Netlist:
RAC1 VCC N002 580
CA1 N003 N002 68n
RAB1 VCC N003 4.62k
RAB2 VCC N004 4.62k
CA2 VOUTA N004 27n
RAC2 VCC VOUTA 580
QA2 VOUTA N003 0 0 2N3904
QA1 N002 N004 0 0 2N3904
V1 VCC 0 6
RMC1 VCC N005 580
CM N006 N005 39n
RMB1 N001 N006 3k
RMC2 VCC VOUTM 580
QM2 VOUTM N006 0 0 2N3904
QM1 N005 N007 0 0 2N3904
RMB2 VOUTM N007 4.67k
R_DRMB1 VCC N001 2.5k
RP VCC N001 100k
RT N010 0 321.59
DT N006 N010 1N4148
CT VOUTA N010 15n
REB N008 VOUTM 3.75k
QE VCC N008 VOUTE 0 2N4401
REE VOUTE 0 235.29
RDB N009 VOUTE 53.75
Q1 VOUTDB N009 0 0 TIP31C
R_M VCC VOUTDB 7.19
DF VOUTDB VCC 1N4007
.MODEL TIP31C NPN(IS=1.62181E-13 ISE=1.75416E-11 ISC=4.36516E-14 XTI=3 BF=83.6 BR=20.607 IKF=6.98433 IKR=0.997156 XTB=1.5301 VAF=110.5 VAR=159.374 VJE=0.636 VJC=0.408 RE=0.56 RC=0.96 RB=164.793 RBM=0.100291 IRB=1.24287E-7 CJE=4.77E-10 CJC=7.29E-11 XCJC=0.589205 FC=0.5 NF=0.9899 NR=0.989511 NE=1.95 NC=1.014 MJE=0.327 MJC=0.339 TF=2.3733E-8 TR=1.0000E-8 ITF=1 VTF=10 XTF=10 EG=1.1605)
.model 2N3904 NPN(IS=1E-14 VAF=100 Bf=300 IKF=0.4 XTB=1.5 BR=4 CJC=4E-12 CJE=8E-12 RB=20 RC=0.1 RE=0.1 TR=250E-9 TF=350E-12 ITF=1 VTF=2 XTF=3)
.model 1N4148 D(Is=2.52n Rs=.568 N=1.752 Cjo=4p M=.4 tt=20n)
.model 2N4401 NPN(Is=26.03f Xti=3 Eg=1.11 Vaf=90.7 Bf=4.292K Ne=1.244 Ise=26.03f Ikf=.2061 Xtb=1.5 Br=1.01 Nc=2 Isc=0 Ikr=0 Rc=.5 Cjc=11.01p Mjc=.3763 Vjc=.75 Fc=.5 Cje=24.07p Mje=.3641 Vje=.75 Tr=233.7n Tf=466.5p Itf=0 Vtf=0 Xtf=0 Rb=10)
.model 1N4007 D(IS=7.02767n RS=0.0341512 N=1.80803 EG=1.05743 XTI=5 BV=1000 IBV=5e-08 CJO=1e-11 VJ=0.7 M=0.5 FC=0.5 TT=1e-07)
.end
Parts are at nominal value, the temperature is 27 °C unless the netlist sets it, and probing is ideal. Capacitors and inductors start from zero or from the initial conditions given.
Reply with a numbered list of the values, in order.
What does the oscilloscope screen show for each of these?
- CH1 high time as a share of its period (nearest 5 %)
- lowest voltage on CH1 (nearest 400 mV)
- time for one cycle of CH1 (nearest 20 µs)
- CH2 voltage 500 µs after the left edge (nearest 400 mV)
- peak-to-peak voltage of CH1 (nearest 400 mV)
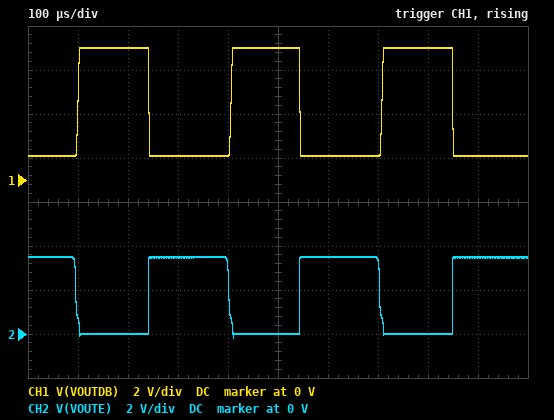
1. 45 %
2. 1.2 V
3. 300 µs
4. 0 V
5. 4.8 V
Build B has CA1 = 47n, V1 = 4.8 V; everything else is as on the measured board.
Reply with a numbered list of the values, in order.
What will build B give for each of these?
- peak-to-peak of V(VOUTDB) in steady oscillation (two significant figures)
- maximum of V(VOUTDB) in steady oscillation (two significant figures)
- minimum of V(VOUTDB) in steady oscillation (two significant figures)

1. 3.9 V
2. 4.8 V
3. 890 mV
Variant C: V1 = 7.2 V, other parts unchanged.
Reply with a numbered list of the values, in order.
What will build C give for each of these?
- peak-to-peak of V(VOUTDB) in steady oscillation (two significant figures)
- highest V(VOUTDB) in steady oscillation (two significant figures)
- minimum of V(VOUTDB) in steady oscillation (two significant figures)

1. 5.9 V
2. 7.2 V
3. 1.3 V
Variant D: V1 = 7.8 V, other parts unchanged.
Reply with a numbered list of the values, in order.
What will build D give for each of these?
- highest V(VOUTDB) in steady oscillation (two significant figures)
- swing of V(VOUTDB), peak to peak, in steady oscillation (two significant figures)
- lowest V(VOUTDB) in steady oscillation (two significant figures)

1. 7.8 V
2. 6.4 V
3. 1.4 V
